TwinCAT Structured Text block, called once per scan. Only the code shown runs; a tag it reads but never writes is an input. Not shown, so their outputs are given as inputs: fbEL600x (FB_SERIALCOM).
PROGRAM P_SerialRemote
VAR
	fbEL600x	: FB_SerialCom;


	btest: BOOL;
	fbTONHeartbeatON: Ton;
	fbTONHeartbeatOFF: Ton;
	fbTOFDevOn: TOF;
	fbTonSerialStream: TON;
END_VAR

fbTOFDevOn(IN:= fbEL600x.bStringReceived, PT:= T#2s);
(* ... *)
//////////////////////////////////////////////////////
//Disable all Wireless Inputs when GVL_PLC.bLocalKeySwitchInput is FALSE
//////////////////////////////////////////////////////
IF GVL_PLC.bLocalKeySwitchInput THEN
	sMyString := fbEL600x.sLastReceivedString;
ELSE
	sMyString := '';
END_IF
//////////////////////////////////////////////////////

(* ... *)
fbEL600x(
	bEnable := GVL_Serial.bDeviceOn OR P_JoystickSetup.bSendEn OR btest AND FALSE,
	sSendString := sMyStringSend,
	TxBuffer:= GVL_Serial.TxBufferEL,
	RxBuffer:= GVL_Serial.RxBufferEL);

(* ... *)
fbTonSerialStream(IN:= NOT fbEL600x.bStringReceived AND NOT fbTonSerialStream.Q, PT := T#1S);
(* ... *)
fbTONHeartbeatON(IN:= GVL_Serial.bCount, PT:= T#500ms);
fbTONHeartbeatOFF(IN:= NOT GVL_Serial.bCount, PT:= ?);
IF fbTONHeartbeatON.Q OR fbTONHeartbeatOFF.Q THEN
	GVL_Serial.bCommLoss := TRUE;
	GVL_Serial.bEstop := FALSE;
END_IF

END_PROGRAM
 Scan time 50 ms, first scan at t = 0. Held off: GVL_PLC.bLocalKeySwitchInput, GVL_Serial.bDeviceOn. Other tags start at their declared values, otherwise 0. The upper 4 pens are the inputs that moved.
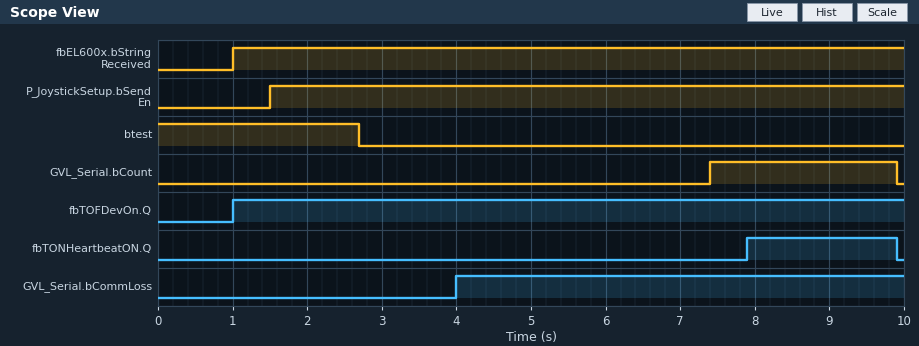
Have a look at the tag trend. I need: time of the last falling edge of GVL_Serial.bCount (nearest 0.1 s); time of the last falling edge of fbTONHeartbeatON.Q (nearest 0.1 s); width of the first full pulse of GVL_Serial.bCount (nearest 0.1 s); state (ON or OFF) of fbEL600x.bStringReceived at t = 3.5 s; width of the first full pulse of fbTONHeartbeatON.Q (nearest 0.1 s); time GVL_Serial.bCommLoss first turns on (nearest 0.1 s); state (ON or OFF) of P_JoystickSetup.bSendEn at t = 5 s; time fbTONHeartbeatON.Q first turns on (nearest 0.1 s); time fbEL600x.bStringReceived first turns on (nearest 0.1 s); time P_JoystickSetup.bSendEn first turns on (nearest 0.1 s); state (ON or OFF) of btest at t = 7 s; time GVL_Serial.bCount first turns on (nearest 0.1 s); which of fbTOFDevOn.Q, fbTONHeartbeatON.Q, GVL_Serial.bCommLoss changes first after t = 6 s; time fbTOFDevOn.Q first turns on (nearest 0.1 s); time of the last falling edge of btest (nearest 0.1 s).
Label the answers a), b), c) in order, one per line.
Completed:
a) 9.9 s
b) 9.9 s
c) 2.5 s
d) ON
e) 2.0 s
f) 4.0 s
g) ON
h) 7.9 s
i) 1.0 s
j) 1.5 s
k) OFF
l) 7.4 s
m) fbTONHeartbeatON.Q
n) 1.0 s
o) 2.7 s
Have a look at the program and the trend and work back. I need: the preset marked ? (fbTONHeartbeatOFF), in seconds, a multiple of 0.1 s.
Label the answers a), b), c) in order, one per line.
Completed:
a) 4.0 s
